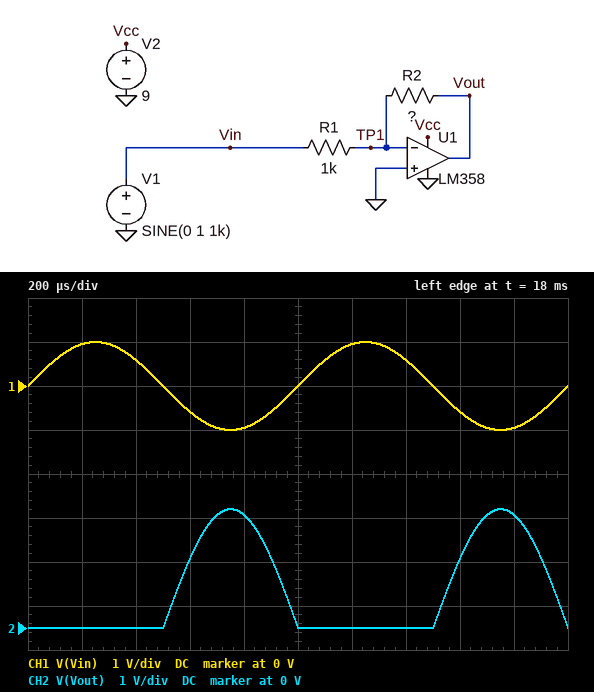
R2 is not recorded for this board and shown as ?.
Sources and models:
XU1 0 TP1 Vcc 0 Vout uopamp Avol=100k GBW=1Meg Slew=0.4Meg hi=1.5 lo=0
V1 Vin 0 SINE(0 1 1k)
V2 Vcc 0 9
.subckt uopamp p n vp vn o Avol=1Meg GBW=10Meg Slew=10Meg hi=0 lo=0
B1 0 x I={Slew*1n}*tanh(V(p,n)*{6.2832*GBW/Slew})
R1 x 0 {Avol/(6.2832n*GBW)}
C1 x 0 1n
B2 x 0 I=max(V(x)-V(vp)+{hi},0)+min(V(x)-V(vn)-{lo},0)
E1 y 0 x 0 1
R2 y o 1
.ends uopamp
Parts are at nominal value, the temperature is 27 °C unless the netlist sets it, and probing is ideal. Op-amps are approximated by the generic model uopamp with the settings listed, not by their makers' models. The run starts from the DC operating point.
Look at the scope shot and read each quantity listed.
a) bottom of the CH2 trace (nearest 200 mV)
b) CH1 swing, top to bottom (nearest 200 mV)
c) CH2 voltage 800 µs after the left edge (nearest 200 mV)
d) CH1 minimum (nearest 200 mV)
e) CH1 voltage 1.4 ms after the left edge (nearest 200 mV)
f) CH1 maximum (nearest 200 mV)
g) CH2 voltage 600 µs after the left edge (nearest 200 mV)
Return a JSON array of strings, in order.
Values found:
["0 V", "2.0 V", "2.6 V", "-1.0 V", "600 mV", "1.0 V", "1.6 V"]
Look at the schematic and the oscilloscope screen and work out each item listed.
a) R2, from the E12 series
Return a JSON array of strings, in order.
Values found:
["2.7 kΩ"]
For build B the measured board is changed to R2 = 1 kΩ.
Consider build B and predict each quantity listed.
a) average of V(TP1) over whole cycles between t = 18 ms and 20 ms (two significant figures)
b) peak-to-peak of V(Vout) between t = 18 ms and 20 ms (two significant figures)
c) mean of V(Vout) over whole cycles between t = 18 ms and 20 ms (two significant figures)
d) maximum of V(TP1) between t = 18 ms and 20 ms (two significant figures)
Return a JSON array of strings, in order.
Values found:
["160 mV", "1.0 V", "320 mV", "500 mV"]
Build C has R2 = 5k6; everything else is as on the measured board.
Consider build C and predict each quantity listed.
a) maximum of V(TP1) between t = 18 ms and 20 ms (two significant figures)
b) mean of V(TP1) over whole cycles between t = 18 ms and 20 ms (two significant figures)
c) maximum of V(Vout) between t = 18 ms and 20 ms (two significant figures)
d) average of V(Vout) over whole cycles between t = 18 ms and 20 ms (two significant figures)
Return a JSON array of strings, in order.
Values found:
["850 mV", "270 mV", "5.6 V", "1.8 V"]
